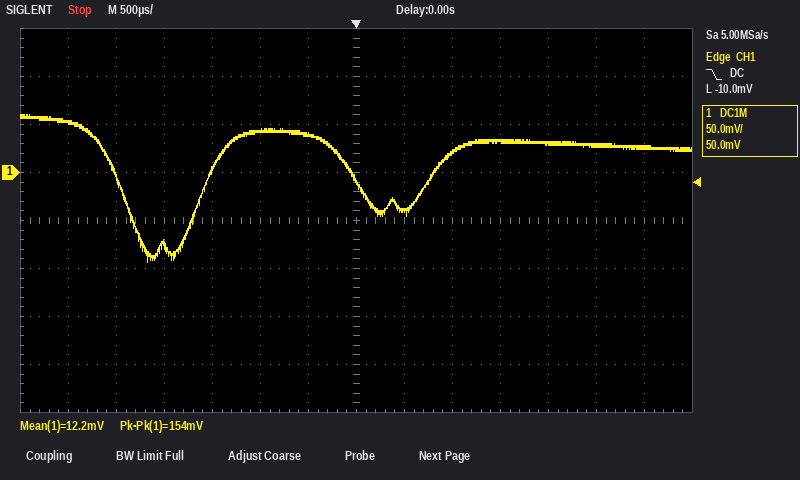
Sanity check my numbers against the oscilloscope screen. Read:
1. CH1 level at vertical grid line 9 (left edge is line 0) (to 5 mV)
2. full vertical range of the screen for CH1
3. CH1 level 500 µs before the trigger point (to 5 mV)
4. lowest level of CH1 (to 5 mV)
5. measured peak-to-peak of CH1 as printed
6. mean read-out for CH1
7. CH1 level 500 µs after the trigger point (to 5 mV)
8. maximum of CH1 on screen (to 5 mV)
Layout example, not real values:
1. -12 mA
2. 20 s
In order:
1. 20 mV
2. 400 mV
3. 40 mV
4. -95 mV
5. 154 mV
6. 12.2 mV
7. -40 mV
8. 60 mV
